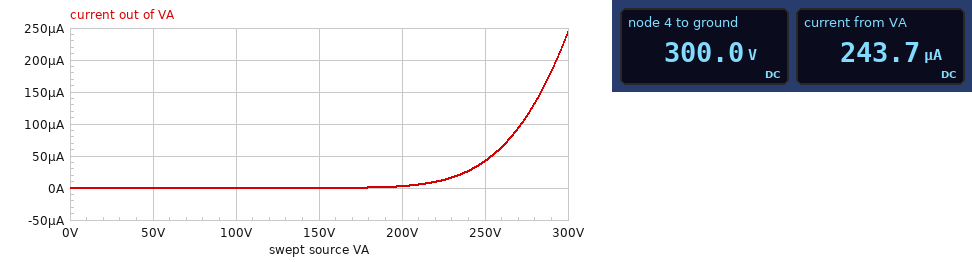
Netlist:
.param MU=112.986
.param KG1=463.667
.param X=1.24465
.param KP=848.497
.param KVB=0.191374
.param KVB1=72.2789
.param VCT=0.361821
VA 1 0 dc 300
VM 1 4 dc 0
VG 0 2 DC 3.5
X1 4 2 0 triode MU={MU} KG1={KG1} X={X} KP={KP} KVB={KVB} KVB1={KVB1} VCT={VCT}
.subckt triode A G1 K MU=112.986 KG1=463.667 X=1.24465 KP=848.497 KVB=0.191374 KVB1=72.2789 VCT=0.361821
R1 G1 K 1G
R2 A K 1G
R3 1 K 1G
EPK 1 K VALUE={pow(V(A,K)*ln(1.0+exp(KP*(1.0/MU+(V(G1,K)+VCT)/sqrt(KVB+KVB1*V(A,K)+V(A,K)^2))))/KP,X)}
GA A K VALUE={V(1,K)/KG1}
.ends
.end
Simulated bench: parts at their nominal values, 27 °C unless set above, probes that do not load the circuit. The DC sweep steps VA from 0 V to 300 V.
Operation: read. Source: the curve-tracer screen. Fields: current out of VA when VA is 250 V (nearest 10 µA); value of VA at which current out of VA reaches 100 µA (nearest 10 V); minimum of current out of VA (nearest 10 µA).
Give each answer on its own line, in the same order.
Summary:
40 µA
270 V
0 A
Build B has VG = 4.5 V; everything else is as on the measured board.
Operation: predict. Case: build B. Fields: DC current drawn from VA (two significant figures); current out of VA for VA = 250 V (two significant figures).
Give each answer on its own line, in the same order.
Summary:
14 µA
1.4 µA
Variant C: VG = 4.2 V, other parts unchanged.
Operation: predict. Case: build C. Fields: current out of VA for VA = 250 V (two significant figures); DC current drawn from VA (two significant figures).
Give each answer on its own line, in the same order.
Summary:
3.6 µA
35 µA
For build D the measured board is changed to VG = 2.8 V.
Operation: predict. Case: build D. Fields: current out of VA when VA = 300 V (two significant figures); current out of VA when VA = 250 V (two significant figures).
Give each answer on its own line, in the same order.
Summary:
1.0 mA
360 µA
